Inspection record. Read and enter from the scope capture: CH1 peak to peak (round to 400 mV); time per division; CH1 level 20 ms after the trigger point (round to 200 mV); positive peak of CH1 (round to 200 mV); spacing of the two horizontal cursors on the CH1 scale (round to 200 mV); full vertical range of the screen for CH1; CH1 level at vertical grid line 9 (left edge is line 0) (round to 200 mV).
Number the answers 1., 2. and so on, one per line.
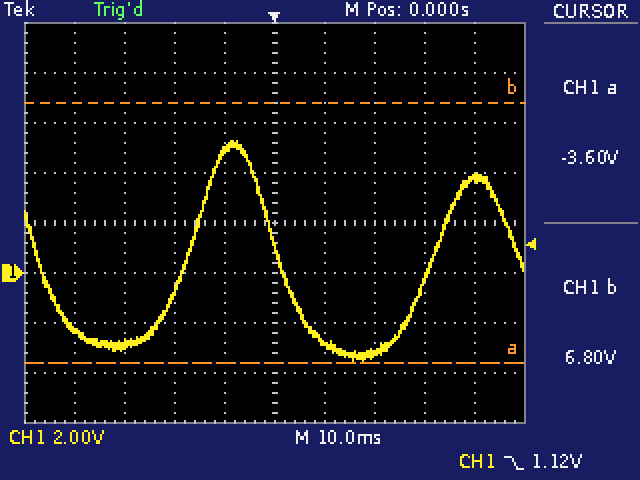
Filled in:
1. 8.8 V
2. 10 ms
3. -3.2 V
4. 5.2 V
5. 10.4 V
6. 16 V
7. 3.8 V
